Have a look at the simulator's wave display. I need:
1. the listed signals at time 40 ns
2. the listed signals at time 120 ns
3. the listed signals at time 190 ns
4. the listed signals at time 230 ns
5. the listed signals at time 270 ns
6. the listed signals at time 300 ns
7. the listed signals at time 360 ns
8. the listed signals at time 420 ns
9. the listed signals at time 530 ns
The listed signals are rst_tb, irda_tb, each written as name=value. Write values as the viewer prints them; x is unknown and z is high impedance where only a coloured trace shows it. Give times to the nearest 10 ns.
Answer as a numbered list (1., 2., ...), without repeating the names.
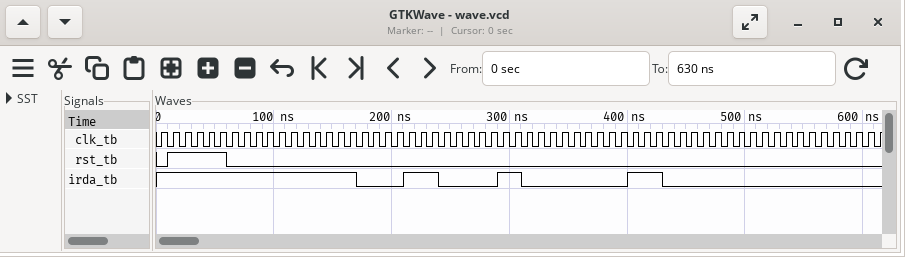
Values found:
1. rst_tb=1, irda_tb=1
2. rst_tb=0, irda_tb=1
3. rst_tb=0, irda_tb=0
4. rst_tb=0, irda_tb=1
5. rst_tb=0, irda_tb=0
6. rst_tb=0, irda_tb=1
7. rst_tb=0, irda_tb=0
8. rst_tb=0, irda_tb=1
9. rst_tb=0, irda_tb=0
